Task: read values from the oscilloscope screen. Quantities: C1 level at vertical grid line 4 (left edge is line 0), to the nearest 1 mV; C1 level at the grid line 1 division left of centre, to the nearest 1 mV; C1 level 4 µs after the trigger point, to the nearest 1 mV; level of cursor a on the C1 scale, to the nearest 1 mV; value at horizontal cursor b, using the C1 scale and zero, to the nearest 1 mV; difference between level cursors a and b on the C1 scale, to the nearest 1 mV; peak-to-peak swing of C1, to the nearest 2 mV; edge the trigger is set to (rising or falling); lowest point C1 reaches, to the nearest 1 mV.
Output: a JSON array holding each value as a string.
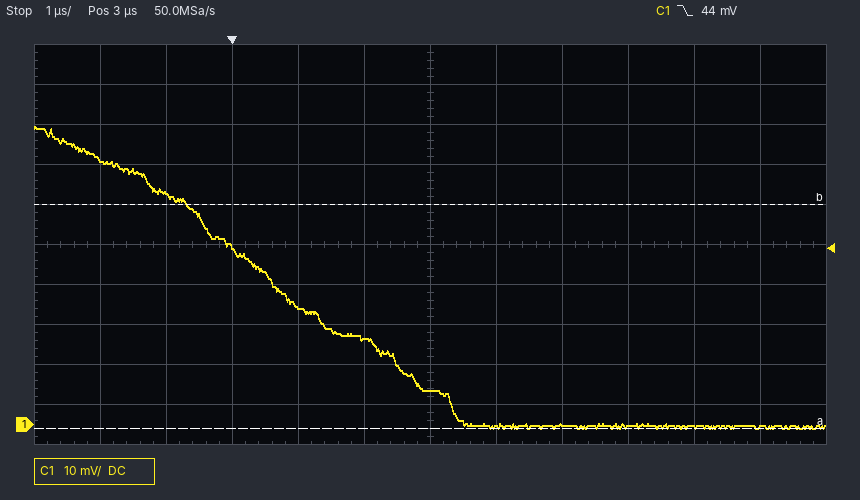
["29 mV", "21 mV", "-1 mV", "-1 mV", "55 mV", "56 mV", "76 mV", "falling", "-1 mV"]
